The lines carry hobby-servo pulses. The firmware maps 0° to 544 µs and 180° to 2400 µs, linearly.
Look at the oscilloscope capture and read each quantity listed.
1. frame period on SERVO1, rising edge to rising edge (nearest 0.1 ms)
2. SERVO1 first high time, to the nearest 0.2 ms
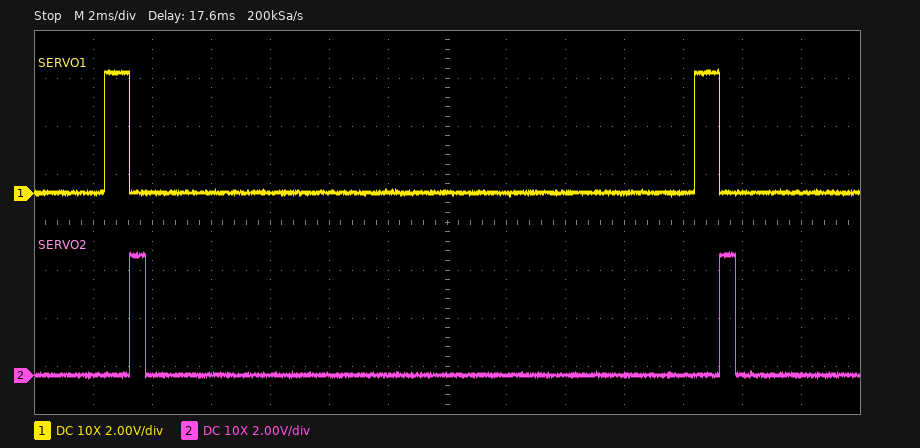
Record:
20.0 ms
0.8 ms
